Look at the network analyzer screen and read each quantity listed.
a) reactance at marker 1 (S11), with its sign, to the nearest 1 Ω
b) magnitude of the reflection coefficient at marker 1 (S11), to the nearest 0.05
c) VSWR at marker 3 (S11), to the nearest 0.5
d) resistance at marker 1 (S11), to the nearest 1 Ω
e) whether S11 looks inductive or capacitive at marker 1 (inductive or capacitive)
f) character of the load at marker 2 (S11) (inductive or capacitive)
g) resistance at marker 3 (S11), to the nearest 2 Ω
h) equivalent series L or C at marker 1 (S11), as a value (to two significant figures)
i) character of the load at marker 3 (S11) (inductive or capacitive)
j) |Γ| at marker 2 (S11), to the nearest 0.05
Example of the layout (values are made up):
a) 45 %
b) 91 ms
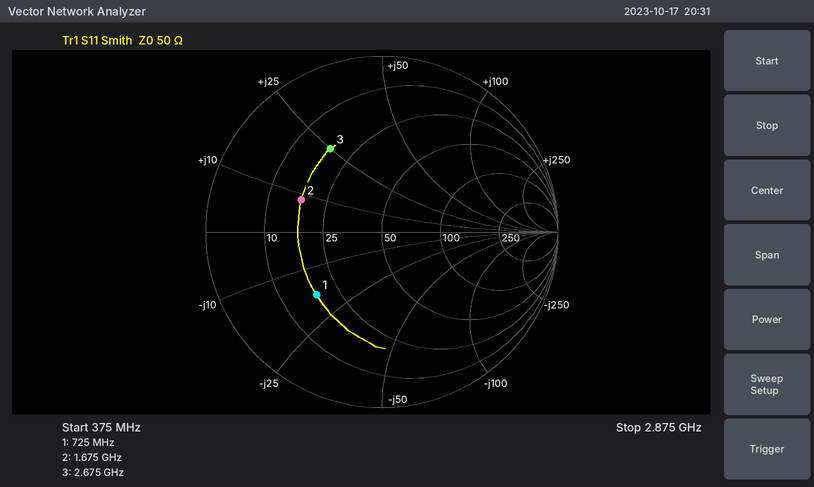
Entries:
a) -18 Ω
b) 0.50
c) 3.5
d) 18 Ω
e) capacitive
f) inductive
g) 18 Ω
h) 12 pF
i) inductive
j) 0.50
